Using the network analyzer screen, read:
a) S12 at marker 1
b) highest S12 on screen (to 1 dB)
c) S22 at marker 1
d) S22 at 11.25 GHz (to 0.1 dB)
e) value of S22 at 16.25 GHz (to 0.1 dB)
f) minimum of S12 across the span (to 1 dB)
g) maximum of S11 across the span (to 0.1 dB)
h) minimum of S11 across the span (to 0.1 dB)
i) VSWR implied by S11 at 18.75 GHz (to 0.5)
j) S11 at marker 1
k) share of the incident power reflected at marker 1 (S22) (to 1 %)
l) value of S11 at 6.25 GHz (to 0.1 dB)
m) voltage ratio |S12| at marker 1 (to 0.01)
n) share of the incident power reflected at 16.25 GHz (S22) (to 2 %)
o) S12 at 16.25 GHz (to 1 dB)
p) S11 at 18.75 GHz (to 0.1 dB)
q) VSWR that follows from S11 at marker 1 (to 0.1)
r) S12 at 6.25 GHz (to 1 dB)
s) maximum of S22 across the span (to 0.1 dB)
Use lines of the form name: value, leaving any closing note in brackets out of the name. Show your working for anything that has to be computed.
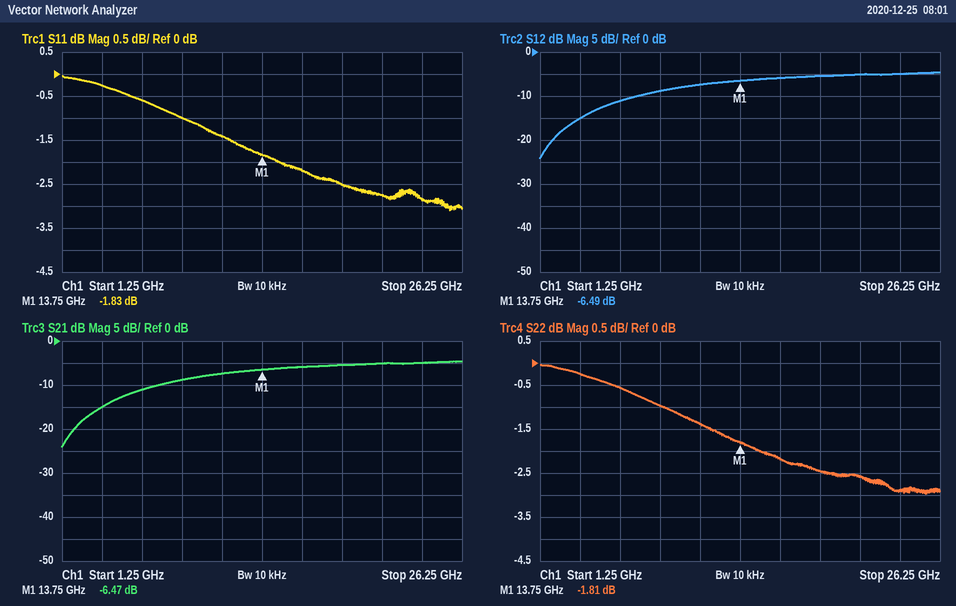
S12 at marker 1: -6.49 dB
highest S12 on screen: -5 dB
S22 at marker 1: -1.81 dB
S22 at 11.25 GHz: -1.4 dB
value of S22 at 16.25 GHz: -2.2 dB
minimum of S12 across the span: -24 dB
maximum of S11 across the span: 0.0 dB
minimum of S11 across the span: -3.1 dB
VSWR implied by S11 at 18.75 GHz: |Γ| = 10^(-2.5/20) = 0.7499; VSWR = (1 + 0.7499)/(1 − 0.7499) ≈ 7.0
S11 at marker 1: -1.83 dB
share of the incident power reflected at marker 1 (S22): 10^(-1.81/10) ≈ 66 %
value of S11 at 6.25 GHz: -0.6 dB
voltage ratio |S12| at marker 1: 10^(-6.49/20) ≈ 0.47
share of the incident power reflected at 16.25 GHz (S22): 10^(-2.2/10) ≈ 60 %
S12 at 16.25 GHz: -6 dB
S11 at 18.75 GHz: -2.5 dB
VSWR that follows from S11 at marker 1: (1 + 0.8100)/(1 − 0.8100) ≈ 9.5
S12 at 6.25 GHz: -11 dB
maximum of S22 across the span: 0.0 dB
